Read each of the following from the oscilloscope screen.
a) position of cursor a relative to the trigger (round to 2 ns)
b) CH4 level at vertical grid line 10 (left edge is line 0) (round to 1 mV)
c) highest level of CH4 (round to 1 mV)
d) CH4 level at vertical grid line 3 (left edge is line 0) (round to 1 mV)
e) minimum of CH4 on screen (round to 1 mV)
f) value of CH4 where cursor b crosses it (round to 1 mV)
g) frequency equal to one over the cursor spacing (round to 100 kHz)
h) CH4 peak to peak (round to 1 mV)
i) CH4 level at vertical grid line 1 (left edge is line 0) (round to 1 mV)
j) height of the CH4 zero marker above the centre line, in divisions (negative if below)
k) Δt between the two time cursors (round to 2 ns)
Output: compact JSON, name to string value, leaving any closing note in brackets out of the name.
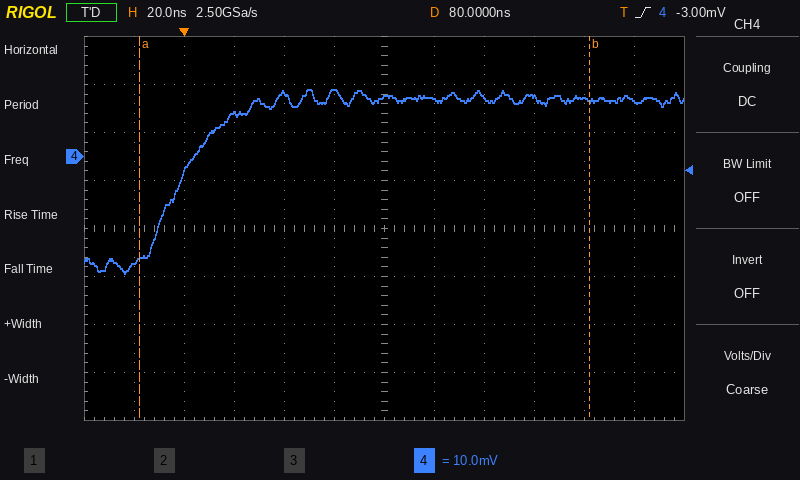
{"position of cursor a relative to the trigger": "-18 ns", "CH4 level at vertical grid line 10 (left edge is line 0)": "12 mV", "highest level of CH4": "14 mV", "CH4 level at vertical grid line 3 (left edge is line 0)": "9 mV", "minimum of CH4 on screen": "-24 mV", "value of CH4 where cursor b crosses it": "12 mV", "frequency equal to one over the cursor spacing": "5.6 MHz", "CH4 peak to peak": "38 mV", "CH4 level at vertical grid line 1 (left edge is line 0)": "-22 mV", "height of the CH4 zero marker above the centre line, in divisions": "+1.5 div", "Δt between the two time cursors": "180 ns"}
